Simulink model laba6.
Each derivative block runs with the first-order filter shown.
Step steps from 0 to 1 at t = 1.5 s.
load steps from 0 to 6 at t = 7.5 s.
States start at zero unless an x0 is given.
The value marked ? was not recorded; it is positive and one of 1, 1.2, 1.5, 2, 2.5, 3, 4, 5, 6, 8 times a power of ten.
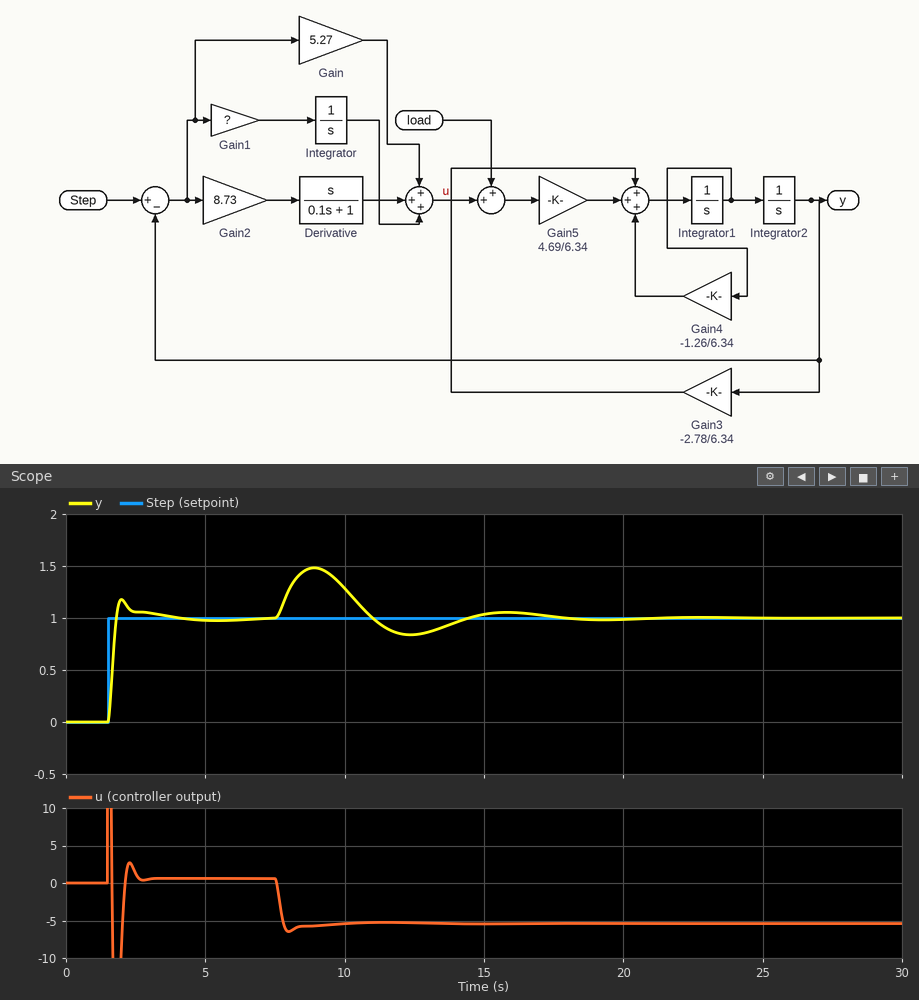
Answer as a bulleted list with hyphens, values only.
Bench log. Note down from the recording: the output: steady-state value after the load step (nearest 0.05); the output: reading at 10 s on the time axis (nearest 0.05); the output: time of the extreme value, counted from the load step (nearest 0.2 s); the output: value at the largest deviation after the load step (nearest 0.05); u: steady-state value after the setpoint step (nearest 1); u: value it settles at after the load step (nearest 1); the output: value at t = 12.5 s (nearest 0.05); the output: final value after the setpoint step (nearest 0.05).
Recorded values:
- 1.00
- 1.30
- 1.4 s
- 1.50
- 1
- -5
- 0.85
- 1.00
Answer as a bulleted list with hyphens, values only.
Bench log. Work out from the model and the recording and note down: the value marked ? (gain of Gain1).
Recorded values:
- 8
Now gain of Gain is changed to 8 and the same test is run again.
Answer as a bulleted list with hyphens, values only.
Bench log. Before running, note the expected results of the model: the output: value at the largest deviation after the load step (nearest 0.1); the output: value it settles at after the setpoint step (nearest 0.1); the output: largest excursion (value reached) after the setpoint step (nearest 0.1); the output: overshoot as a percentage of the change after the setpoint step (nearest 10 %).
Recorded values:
- 1.4
- 1.0
- 1.2
- 20 %
